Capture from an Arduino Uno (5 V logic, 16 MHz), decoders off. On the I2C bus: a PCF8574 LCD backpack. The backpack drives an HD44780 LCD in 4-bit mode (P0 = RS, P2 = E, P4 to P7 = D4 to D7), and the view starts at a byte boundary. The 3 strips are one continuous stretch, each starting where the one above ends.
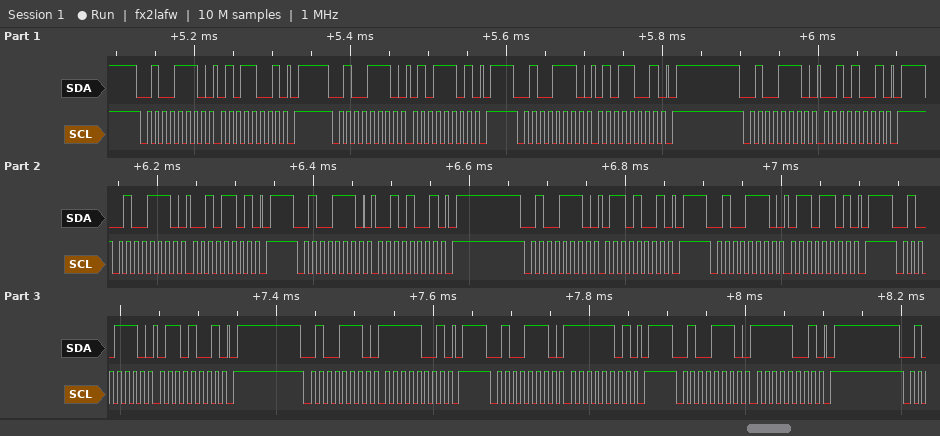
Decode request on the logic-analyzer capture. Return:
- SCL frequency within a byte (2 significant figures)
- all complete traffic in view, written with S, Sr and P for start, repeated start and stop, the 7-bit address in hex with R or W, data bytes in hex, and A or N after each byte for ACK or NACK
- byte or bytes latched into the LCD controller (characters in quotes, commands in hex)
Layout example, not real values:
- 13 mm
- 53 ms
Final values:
- 100 kHz
- S 27W A 59 A P S 27W A 5D A P S 27W A 59 A P S 27W A 29 A P S 27W A 2D A P S 27W A 29 A P S 27W A 69 A P S 27W A 6D A P S 27W A 69 A P S 27W A F9 A P S 27W A FD A P S 27W A F9 A P
- 'R' 'o'
